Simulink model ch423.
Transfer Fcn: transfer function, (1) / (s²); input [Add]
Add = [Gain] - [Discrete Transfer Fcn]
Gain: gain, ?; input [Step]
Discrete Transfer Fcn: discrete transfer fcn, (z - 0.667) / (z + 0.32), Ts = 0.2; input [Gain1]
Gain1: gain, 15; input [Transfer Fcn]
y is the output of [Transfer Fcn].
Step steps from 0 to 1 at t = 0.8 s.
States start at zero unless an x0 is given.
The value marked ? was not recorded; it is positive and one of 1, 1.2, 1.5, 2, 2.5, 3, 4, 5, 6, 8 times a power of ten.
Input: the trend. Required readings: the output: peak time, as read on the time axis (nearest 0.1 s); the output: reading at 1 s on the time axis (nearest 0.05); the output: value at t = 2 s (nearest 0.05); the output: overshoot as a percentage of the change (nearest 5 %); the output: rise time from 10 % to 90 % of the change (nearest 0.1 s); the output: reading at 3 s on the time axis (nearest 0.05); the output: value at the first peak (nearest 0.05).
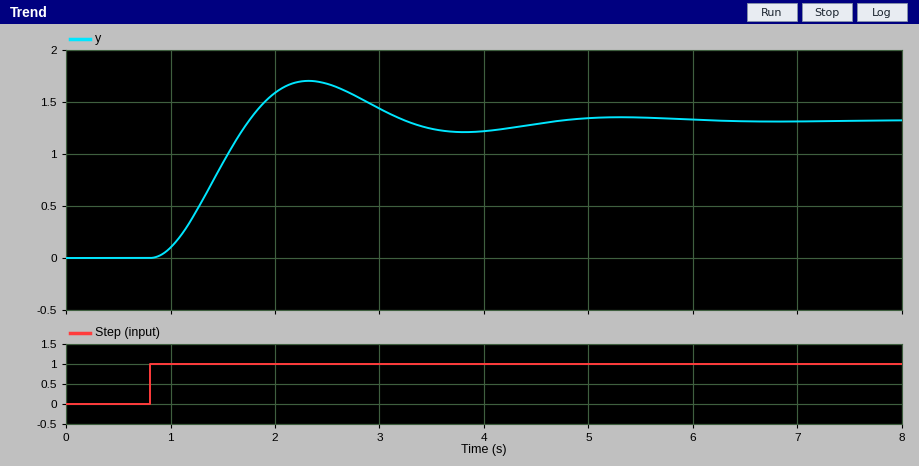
2.3 s
0.10
1.60
30 %
0.6 s
1.45
1.70
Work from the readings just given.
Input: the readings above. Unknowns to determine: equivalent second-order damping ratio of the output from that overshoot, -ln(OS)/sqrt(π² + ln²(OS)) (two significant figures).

0.36
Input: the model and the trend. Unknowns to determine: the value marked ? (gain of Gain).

5
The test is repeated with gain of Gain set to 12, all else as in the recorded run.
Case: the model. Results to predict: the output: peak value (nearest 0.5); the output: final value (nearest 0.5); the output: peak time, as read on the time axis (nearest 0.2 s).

4.0
3.0
2.4 s
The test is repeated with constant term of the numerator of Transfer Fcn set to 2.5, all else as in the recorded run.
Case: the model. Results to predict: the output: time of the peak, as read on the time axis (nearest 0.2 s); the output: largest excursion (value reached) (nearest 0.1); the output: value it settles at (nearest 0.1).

1.6 s
1.4
1.3
